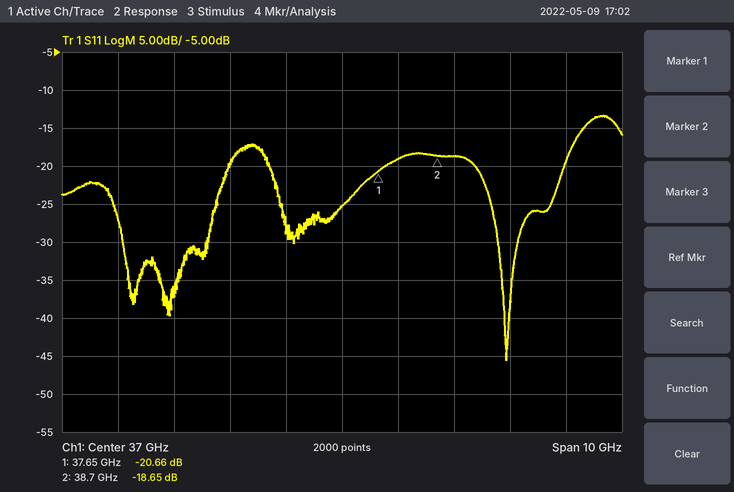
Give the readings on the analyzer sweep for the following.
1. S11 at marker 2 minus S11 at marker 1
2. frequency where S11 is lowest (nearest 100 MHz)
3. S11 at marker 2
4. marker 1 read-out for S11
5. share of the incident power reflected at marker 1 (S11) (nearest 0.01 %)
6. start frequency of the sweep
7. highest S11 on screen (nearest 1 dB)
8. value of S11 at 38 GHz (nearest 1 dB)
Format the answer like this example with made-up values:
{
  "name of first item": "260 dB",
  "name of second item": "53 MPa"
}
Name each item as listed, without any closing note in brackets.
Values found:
{
  "S11 at marker 2 minus S11 at marker 1": "2.01 dB",
  "frequency where S11 is lowest": "39.9 GHz",
  "S11 at marker 2": "-18.65 dB",
  "marker 1 read-out for S11": "-20.66 dB",
  "share of the incident power reflected at marker 1 (S11)": "0.86 %",
  "start frequency of the sweep": "32 GHz",
  "highest S11 on screen": "-13 dB",
  "value of S11 at 38 GHz": "-19 dB"
}
